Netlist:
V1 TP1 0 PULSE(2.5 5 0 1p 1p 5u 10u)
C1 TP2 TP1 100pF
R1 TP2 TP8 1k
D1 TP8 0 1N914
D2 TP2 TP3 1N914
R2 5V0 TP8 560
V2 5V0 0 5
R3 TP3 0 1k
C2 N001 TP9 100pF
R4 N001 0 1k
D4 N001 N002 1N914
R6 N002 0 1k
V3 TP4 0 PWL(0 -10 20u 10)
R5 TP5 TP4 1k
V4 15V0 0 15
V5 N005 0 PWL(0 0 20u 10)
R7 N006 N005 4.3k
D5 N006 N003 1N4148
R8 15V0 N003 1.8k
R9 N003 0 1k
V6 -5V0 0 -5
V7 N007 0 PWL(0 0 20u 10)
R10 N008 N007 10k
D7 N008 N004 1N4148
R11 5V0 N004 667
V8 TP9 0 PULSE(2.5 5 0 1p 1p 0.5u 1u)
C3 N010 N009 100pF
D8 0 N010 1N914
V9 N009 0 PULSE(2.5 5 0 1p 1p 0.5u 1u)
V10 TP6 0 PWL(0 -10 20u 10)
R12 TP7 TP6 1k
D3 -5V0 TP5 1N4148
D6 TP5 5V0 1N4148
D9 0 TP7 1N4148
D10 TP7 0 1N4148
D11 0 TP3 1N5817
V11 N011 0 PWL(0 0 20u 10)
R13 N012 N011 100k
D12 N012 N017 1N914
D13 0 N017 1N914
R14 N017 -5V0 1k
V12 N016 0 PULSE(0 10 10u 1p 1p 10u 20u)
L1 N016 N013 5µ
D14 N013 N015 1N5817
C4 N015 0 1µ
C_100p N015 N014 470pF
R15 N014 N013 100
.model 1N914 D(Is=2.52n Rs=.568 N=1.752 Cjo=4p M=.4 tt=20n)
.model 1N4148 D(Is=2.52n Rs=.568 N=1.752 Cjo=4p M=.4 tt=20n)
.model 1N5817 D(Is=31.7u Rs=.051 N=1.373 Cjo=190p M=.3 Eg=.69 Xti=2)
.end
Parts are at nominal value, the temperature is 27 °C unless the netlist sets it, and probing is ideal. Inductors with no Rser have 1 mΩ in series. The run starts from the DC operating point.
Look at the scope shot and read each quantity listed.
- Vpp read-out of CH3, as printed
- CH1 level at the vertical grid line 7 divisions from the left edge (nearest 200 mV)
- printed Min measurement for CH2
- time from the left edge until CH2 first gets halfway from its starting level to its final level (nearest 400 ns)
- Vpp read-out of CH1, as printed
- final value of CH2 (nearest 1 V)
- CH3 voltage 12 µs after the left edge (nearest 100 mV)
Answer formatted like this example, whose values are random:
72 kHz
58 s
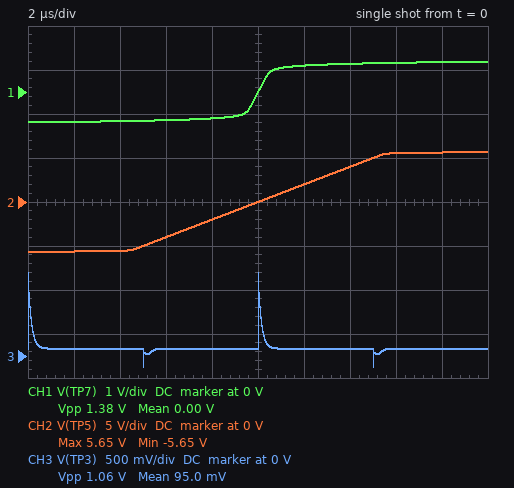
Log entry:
1.06 V
600 mV
-5.65 V
10.0 µs
1.38 V
6 V
100 mV
